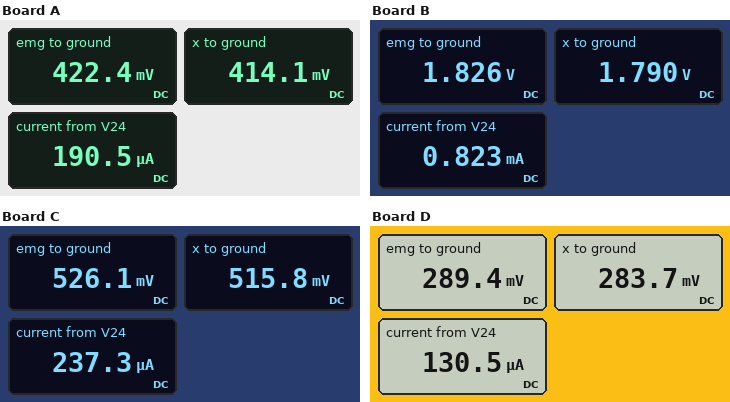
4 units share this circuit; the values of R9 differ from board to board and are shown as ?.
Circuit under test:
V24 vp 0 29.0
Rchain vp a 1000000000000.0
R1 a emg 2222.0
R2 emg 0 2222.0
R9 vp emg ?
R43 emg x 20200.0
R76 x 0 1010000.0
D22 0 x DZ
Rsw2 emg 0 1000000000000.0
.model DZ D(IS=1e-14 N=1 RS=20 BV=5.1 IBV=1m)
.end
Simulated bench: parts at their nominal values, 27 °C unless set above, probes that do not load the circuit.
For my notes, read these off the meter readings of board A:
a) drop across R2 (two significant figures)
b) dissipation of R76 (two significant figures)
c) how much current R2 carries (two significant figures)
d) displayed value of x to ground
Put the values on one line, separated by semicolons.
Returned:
420 mV; 170 nW; 190 µA; 414.1 mV
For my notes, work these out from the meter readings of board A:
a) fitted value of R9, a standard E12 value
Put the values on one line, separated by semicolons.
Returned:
150 kΩ
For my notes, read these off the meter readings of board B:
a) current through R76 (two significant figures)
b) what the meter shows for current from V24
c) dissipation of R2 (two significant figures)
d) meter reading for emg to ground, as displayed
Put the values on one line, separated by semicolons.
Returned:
1.8 µA; 0.823 mA; 1.5 mW; 1.826 V
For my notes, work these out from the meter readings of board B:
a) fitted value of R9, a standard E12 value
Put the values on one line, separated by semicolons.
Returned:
33 kΩ
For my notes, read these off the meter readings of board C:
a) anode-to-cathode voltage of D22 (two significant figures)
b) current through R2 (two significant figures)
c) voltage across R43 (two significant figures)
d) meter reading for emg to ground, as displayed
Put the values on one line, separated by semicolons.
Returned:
-520 mV; 240 µA; 10 mV; 526.1 mV
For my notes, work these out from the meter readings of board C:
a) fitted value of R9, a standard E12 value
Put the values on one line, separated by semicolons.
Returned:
120 kΩ
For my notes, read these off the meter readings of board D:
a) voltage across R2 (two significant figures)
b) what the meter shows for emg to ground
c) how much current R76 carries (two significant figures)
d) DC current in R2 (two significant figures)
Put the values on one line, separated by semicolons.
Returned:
290 mV; 289.4 mV; 280 nA; 130 µA
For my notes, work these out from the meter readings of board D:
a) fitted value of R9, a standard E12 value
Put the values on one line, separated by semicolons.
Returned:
220 kΩ
